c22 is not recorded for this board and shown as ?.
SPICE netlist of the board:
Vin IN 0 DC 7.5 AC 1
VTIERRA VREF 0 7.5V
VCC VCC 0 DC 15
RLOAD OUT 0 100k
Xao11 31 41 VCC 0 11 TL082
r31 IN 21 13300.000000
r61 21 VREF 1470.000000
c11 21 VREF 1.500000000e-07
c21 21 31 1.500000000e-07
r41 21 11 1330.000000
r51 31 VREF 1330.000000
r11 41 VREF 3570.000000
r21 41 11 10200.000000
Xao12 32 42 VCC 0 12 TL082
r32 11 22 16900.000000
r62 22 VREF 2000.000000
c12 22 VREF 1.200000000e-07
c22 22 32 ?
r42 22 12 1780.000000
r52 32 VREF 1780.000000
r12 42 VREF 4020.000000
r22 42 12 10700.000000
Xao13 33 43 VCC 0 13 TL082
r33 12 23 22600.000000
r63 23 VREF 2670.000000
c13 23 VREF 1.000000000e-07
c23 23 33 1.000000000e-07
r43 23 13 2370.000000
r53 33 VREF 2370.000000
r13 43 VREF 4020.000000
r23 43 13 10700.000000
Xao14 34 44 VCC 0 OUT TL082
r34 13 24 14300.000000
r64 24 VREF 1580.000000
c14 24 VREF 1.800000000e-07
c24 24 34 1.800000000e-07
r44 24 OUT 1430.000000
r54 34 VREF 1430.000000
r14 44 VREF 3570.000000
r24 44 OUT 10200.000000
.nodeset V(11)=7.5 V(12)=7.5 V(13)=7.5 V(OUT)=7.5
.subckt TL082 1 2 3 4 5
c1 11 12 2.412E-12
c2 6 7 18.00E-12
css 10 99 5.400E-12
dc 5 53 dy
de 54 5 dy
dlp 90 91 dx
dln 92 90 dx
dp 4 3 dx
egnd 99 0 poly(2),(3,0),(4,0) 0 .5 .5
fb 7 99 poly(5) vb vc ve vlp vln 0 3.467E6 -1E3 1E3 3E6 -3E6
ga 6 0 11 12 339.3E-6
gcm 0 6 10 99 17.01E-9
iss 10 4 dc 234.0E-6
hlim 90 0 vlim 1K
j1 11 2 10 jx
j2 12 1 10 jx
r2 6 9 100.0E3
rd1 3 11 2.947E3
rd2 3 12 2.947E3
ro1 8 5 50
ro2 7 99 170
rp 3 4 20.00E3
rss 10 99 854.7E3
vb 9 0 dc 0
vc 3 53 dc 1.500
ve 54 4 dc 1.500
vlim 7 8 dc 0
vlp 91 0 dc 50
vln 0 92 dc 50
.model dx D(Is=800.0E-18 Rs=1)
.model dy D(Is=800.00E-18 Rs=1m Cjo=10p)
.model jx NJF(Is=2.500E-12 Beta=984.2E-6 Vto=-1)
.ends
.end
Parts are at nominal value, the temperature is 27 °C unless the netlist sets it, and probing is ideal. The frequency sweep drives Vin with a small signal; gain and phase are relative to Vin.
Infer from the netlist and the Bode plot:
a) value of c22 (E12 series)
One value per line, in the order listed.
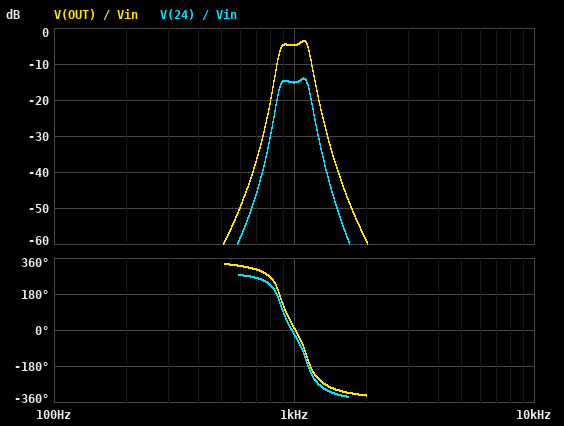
100 nF
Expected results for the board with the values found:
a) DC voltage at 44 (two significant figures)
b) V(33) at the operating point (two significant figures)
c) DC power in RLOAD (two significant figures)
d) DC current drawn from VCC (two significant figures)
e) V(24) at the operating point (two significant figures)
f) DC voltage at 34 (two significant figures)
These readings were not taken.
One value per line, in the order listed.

7.5 V
7.5 V
560 µW
3.9 mA
7.5 V
7.5 V
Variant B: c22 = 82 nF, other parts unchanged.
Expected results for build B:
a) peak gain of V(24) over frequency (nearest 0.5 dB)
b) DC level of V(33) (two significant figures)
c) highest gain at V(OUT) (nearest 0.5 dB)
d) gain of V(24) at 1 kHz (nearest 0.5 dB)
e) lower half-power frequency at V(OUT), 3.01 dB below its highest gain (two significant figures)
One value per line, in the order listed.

-18.5 dB
7.5 V
-8.0 dB
-19.5 dB
860 Hz
